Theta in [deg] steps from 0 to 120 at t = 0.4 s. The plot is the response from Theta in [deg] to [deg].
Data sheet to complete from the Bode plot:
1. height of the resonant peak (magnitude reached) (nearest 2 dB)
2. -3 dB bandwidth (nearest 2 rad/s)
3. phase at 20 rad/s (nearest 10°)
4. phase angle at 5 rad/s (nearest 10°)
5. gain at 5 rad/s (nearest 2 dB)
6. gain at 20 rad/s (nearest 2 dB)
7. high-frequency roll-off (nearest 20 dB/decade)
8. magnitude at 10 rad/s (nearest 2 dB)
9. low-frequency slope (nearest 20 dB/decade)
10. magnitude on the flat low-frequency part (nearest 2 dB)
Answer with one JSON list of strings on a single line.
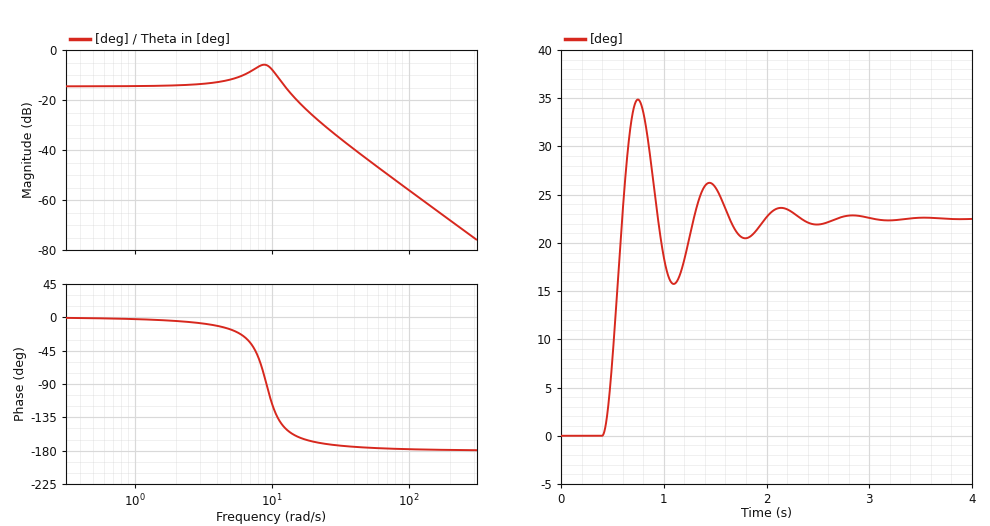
["-6 dB", "14 rad/s", "-170°", "-20°", "-12 dB", "-26 dB", "-40 dB/decade", "-8 dB", "0 dB/decade", "-14 dB"]
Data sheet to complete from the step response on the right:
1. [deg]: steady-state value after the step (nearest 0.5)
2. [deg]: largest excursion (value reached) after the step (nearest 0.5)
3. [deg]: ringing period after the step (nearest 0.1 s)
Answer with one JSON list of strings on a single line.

["22.5", "35.0", "0.7 s"]
